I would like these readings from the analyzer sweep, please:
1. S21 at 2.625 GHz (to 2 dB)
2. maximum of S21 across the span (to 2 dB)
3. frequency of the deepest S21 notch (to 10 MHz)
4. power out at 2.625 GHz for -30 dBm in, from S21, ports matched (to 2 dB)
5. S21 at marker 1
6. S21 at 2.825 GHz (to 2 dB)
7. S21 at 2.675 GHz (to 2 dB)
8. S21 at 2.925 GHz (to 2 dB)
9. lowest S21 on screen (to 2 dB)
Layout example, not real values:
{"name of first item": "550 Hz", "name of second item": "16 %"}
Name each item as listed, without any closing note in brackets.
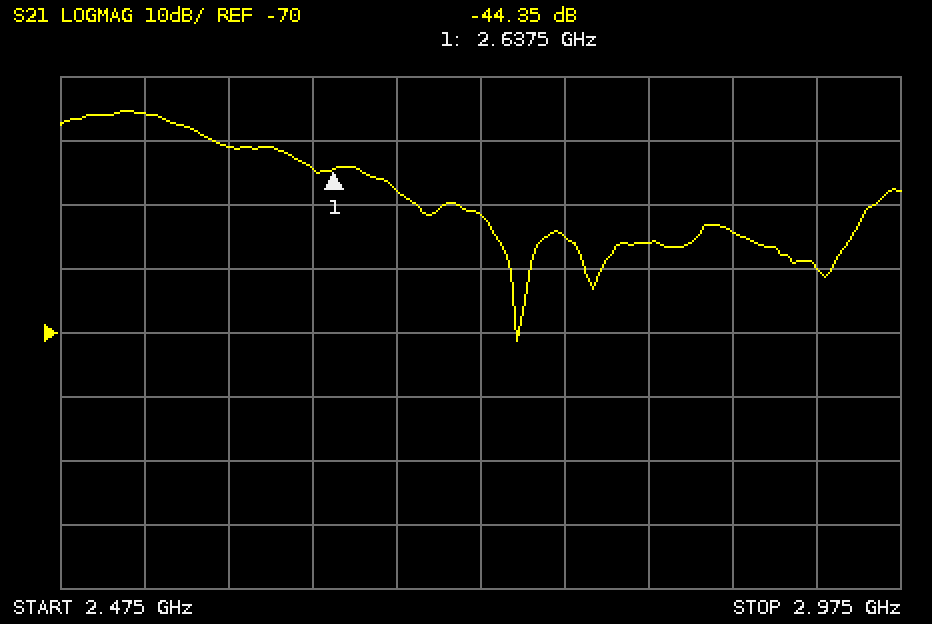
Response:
{"S21 at 2.625 GHz": "-44 dB", "maximum of S21 across the span": "-36 dB", "frequency of the deepest S21 notch": "2.75 GHz", "power out at 2.625 GHz for -30 dBm in, from S21, ports matched": "-74 dBm", "S21 at marker 1": "-44.35 dB", "S21 at 2.825 GHz": "-56 dB", "S21 at 2.675 GHz": "-48 dB", "S21 at 2.925 GHz": "-60 dB", "lowest S21 on screen": "-72 dB"}
